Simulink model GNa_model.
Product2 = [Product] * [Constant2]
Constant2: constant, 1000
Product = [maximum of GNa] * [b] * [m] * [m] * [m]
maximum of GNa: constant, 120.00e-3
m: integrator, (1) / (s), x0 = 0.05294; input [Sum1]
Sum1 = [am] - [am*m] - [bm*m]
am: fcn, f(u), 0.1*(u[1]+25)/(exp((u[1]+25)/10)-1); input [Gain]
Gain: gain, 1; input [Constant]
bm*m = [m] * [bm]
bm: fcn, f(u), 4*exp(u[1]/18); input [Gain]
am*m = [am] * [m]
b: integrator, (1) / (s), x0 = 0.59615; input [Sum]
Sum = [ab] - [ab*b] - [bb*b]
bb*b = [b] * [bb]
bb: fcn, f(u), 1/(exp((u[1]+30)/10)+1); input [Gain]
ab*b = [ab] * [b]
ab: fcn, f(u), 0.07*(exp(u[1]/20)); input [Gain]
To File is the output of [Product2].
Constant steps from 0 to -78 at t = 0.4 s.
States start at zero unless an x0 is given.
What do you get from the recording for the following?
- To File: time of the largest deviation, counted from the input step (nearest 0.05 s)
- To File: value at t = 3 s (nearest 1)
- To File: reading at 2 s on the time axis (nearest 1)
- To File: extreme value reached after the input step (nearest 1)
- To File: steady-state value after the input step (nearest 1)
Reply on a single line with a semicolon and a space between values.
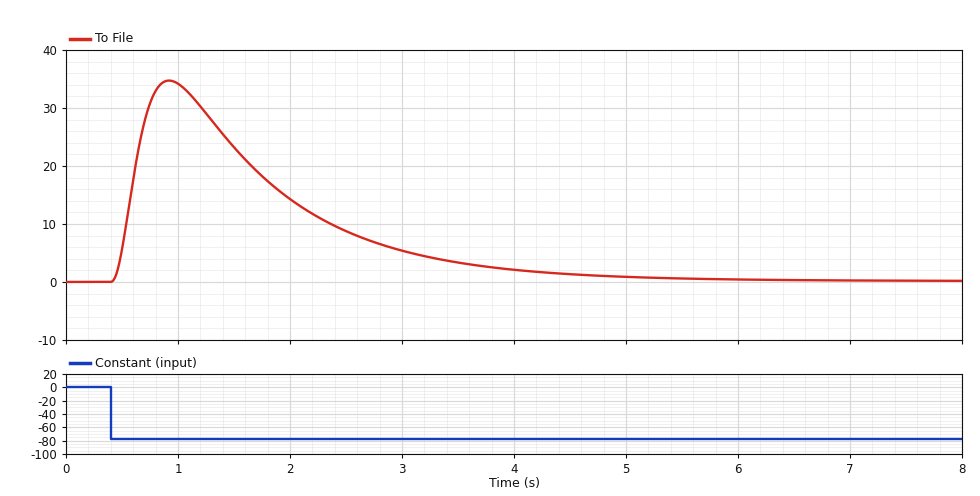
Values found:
0.50 s; 5; 14; 35; 0
